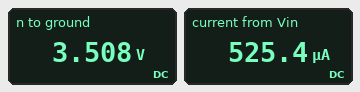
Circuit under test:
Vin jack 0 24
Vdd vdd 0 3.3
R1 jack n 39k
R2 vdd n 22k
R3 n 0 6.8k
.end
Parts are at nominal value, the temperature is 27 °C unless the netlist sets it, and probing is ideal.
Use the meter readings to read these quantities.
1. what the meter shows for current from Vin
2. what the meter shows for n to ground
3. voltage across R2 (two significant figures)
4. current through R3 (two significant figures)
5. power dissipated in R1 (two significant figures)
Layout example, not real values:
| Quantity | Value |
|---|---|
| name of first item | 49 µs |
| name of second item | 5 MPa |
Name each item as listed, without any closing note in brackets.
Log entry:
| Quantity | Value |
|---|---|
| what the meter shows for current from Vin | 525.4 µA |
| what the meter shows for n to ground | 3.508 V |
| voltage across R2 | 210 mV |
| current through R3 | 520 µA |
| power dissipated in R1 | 11 mW |
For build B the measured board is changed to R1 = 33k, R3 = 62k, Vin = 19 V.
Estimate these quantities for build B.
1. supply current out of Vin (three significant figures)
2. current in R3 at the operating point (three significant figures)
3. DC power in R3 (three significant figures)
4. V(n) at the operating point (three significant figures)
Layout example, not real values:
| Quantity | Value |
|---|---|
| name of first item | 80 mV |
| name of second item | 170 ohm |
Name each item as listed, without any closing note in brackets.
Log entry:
| Quantity | Value |
|---|---|
| supply current out of Vin | 336 µA |
| current in R3 at the operating point | 127 µA |
| DC power in R3 | 1.01 mW |
| V(n) at the operating point | 7.90 V |
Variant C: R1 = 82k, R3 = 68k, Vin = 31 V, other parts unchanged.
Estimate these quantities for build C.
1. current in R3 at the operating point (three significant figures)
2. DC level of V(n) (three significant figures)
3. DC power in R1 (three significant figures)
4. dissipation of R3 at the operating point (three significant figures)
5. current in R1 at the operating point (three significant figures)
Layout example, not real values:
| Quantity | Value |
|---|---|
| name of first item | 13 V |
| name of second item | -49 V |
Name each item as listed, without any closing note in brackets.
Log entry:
| Quantity | Value |
|---|---|
| current in R3 at the operating point | 107 µA |
| DC level of V(n) | 7.30 V |
| DC power in R1 | 6.85 mW |
| dissipation of R3 at the operating point | 783 µW |
| current in R1 at the operating point | 289 µA |
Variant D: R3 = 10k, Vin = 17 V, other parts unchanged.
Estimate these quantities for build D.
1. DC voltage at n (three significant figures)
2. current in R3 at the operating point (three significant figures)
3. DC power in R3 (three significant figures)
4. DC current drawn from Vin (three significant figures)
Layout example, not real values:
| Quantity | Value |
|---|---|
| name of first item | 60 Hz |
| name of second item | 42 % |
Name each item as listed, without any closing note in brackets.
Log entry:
| Quantity | Value |
|---|---|
| DC voltage at n | 3.42 V |
| current in R3 at the operating point | 342 µA |
| DC power in R3 | 1.17 mW |
| DC current drawn from Vin | 348 µA |
